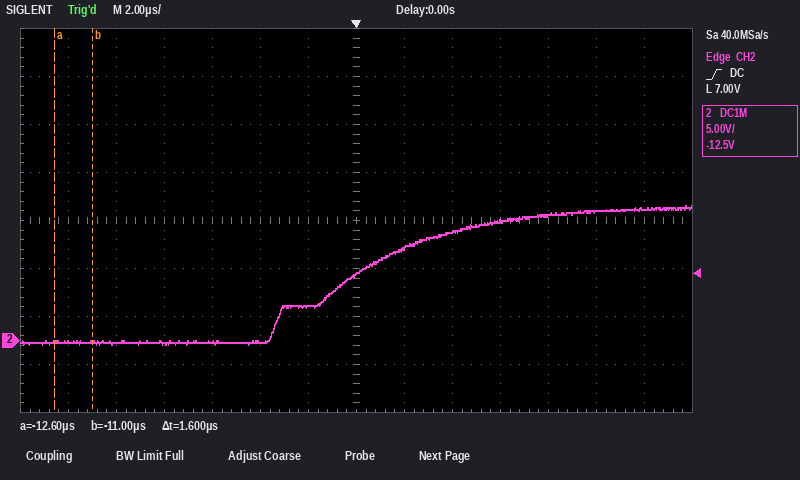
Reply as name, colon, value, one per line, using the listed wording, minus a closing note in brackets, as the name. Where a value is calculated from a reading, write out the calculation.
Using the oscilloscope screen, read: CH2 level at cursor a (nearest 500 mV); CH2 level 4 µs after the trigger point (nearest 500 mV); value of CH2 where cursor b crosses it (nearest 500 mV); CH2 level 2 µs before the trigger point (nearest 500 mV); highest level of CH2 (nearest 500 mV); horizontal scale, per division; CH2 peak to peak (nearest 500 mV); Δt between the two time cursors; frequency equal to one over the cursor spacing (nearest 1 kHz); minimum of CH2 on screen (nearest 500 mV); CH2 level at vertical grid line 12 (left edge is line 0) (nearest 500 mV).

CH2 level at cursor a: 0.0 V
CH2 level 4 µs after the trigger point: 11.5 V
value of CH2 where cursor b crosses it: 0.0 V
CH2 level 2 µs before the trigger point: 3.5 V
highest level of CH2: 14.0 V
horizontal scale, per division: 2 µs
CH2 peak to peak: 14.0 V − (-500 mV) = 14.5 V
Δt between the two time cursors: 1.6 µs
frequency equal to one over the cursor spacing: 1 / 1.6 µs ≈ 625 kHz
minimum of CH2 on screen: -500 mV
CH2 level at vertical grid line 12 (left edge is line 0): 13.5 V
